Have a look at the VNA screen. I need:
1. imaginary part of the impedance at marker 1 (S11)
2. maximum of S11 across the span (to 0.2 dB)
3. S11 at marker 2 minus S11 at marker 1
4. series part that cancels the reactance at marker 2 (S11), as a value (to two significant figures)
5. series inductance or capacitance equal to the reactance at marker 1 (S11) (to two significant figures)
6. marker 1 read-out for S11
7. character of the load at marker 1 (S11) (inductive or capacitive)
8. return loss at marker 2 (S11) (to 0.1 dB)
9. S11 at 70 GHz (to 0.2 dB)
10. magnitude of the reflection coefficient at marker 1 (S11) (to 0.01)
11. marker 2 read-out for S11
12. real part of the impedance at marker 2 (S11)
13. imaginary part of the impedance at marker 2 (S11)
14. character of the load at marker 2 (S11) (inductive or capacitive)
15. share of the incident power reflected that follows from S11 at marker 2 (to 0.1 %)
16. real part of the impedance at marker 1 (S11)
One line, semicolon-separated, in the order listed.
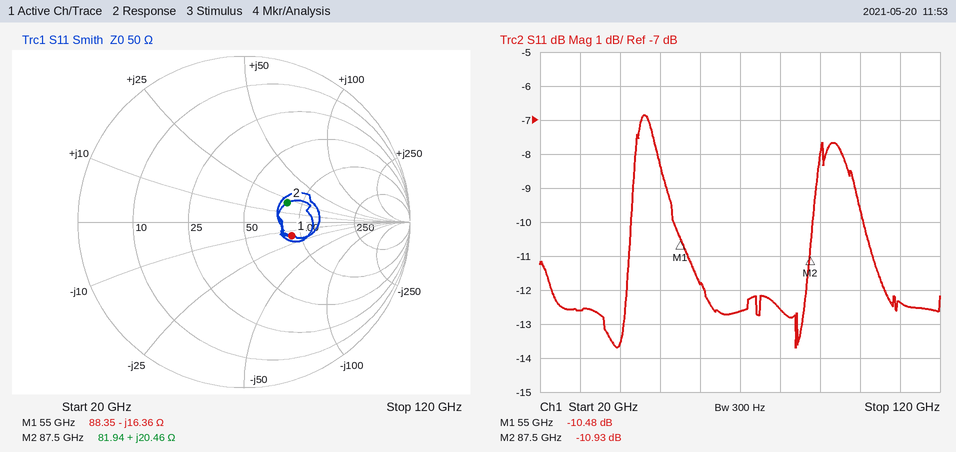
-16.36 Ω; -6.8 dB; -0.45 dB; 89 fF; 180 fF; -10.48 dB; capacitive; 10.9 dB; -12.6 dB; 0.30; -10.93 dB; 81.94 Ω; +20.46 Ω; inductive; 8.1 %; 88.35 Ω
